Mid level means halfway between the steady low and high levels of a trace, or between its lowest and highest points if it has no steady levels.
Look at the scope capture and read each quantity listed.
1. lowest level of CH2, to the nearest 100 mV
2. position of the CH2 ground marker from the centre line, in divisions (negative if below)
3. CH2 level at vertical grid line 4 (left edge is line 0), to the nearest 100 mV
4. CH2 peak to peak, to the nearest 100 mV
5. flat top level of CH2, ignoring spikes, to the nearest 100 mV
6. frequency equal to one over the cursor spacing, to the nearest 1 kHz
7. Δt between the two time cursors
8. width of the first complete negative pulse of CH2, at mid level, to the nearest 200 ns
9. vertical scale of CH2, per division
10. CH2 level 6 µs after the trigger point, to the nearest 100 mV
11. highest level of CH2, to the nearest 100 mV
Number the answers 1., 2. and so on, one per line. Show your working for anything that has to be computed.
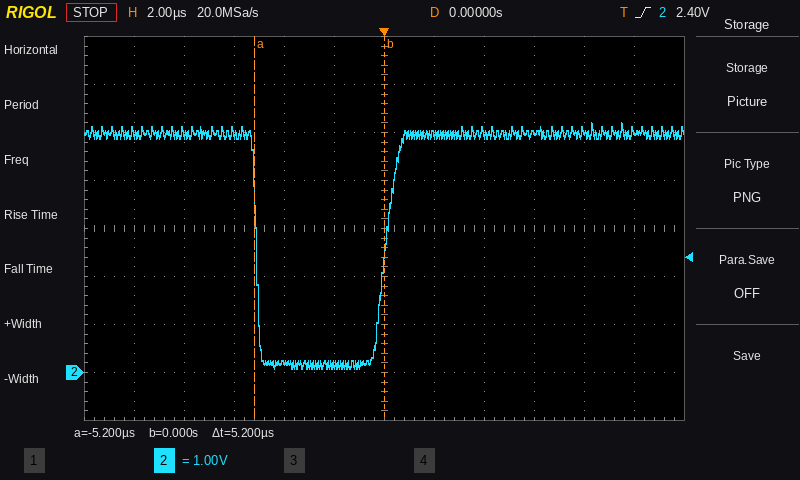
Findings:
1. 100 mV
2. -3.0 div
3. 200 mV
4. 5.2 V − (100 mV) = 5.1 V
5. 5.0 V
6. 1 / 5.2 µs ≈ 192 kHz
7. 5.2 µs
8. 5.2 µs
9. 1 V
10. 5.0 V
11. 5.2 V
